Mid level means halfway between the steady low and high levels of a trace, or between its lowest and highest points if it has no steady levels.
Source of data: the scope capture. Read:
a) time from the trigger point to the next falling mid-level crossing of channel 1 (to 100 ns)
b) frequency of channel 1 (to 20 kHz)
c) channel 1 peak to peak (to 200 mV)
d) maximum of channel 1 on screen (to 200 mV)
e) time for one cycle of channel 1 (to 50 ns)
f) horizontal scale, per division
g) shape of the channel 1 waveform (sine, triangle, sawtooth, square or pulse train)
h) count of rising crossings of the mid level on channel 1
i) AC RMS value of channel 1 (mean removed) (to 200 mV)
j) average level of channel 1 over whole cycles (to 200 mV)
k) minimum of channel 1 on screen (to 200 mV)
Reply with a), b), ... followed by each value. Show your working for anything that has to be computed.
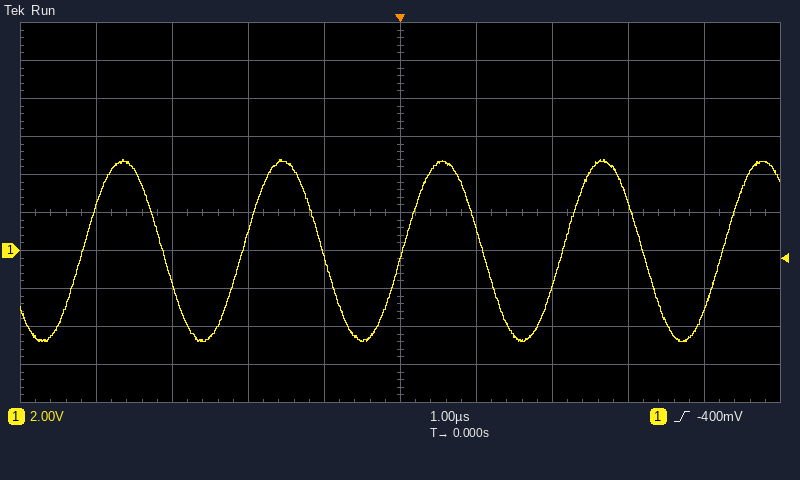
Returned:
a) 1.1 µs
b) 1 / 2.10 µs ≈ 476 kHz, so 480 kHz to the nearest 20 kHz
c) 4.8 V − (-4.8 V) = 9.6 V
d) 4.8 V
e) 2.10 µs
f) 1 µs
g) sine
h) 5
i) 9.6 V / (2√2) ≈ 3.4 V
j) (4.8 V + (-4.8 V)) / 2 ≈ 0.0 V
k) -4.8 V
